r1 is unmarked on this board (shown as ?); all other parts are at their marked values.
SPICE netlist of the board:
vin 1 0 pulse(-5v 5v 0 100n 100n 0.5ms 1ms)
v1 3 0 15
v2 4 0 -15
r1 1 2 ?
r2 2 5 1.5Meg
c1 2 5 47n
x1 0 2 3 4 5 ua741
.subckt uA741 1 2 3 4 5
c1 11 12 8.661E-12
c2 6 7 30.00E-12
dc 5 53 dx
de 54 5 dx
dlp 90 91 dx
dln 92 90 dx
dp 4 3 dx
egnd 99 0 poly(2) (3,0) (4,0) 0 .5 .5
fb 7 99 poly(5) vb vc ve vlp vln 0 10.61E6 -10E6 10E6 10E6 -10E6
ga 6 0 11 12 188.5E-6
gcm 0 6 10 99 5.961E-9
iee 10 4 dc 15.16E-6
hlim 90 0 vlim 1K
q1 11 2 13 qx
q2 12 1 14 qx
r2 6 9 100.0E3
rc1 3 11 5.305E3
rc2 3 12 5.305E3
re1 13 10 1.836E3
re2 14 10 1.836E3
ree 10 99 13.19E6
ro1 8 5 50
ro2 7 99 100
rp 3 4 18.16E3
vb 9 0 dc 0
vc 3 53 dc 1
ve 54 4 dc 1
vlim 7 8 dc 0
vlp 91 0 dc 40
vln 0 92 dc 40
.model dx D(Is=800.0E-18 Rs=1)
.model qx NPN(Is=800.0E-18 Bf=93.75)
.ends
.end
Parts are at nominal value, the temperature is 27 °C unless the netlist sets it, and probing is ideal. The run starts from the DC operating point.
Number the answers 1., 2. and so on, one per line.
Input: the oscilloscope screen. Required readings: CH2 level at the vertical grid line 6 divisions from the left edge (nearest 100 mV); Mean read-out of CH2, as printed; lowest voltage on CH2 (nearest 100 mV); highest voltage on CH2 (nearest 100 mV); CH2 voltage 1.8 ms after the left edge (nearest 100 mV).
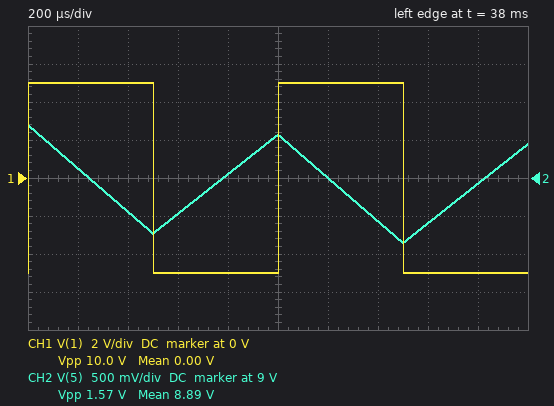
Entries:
1. 9.0 V
2. 8.89 V
3. 8.1 V
4. 9.7 V
5. 8.9 V
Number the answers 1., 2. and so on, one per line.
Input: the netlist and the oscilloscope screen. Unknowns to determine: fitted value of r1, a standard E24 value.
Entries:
1. 39 kΩ
